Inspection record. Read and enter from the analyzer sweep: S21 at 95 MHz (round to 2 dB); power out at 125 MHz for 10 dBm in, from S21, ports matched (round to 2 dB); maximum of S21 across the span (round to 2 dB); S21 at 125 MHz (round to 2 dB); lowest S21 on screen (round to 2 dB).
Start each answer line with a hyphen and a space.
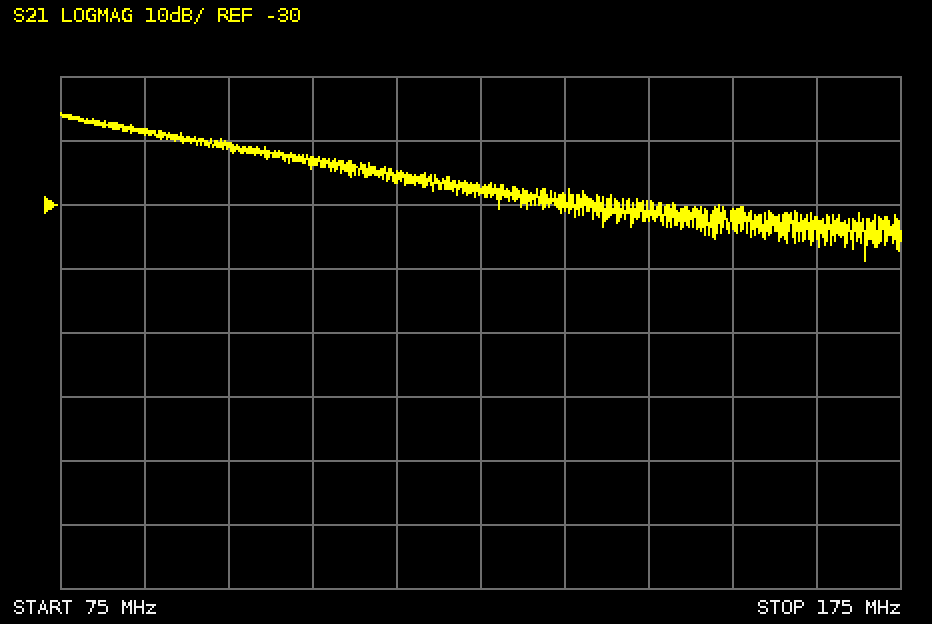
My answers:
- -20 dB
- -18 dBm
- -16 dB
- -28 dB
- -38 dB
